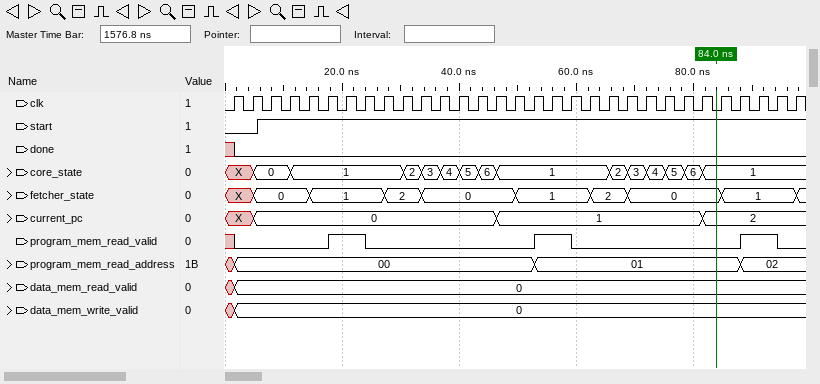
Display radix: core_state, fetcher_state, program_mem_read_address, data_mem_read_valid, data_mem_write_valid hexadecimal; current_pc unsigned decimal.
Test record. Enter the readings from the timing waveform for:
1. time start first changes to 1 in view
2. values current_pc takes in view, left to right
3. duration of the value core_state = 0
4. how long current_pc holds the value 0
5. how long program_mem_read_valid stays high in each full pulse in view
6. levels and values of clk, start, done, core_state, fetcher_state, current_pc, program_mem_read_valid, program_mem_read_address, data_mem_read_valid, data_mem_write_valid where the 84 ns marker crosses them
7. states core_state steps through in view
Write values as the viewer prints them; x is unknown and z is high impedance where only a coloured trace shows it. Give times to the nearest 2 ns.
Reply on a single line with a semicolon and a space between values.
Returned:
6 ns; X, 0, 1, 2; 6 ns; 42 ns; 6 ns, 6 ns, 6 ns; clk=0, start=1, done=0, core_state=1, fetcher_state=0, current_pc=2, program_mem_read_valid=0, program_mem_read_address=01, data_mem_read_valid=0, data_mem_write_valid=0; X, 0, 1, 2, 3, 4, 5, 6, 1, 2, 3, 4, 5, 6, 1
